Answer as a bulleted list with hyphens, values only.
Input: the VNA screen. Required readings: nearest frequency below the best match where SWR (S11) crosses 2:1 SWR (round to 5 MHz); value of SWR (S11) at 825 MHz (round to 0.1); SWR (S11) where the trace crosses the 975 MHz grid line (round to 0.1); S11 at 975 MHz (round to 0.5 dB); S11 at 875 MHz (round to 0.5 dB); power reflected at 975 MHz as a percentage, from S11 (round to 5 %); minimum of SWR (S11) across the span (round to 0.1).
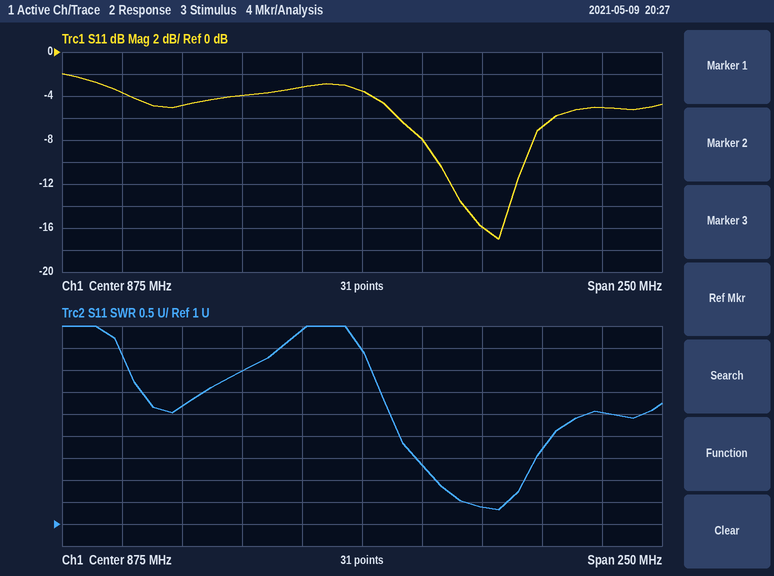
- 905 MHz
- 4.5
- 3.5
- -5.0 dB
- -3.5 dB
- 30 %
- 1.3
